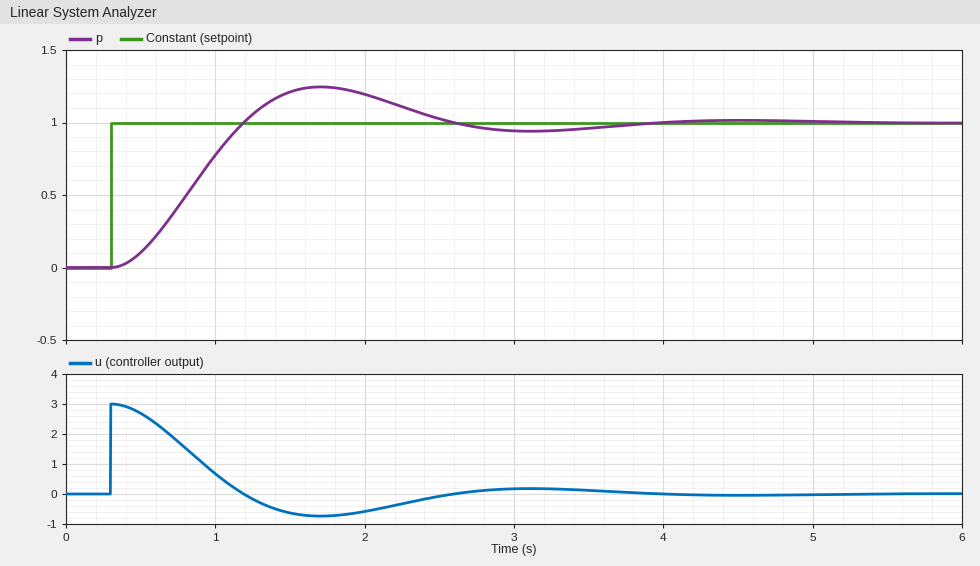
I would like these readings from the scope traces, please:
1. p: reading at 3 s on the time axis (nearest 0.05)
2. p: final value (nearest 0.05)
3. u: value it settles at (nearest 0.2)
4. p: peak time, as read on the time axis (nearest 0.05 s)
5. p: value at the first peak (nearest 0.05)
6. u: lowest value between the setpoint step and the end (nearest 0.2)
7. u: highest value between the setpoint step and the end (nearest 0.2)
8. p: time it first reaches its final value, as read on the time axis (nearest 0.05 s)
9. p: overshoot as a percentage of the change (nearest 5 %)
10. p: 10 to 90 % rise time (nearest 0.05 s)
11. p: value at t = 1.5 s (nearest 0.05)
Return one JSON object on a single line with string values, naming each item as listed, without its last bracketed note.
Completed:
{"p: reading at 3 s on the time axis": "0.95", "p: final value": "1.00", "u: value it settles at": "0.0", "p: peak time, as read on the time axis": "1.70 s", "p: value at the first peak": "1.25", "u: lowest value between the setpoint step and the end": "-0.8", "u: highest value between the setpoint step and the end": "3.0", "p: time it first reaches its final value, as read on the time axis": "1.20 s", "p: overshoot as a percentage of the change": "25 %", "p: 10 to 90 % rise time": "0.60 s", "p: value at t = 1.5 s": "1.20"}
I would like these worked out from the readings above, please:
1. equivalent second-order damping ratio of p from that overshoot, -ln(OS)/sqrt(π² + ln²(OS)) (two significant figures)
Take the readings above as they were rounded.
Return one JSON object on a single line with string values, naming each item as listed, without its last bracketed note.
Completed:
{"equivalent second-order damping ratio of p from that overshoot, -ln(OS)/sqrt(π² + ln²(OS))": "0.40"}
